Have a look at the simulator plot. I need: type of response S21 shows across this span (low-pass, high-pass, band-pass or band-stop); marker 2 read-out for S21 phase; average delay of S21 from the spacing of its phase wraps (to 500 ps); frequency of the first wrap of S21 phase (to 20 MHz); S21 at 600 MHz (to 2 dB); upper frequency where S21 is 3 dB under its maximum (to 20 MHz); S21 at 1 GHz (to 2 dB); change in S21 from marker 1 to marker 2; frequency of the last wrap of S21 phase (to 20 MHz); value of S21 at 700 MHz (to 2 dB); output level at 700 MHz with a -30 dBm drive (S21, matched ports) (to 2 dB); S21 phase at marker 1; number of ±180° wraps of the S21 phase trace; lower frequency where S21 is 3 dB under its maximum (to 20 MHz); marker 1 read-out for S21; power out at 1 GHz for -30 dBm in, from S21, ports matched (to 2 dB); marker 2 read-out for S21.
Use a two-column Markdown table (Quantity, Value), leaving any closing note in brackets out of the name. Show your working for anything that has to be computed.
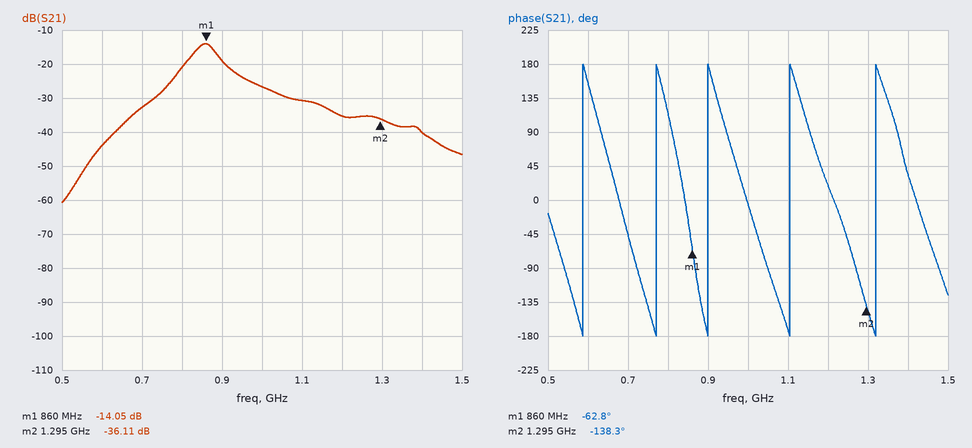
| Quantity | Value |
|---|---|
| type of response S21 shows across this span | band-pass |
| marker 2 read-out for S21 phase | -138.3° |
| average delay of S21 from the spacing of its phase wraps | 4 cycles / (1.32 GHz − 580 MHz) ≈ 5.41 ns, so 5.5 ns to the nearest 500 ps |
| frequency of the first wrap of S21 phase | 580 MHz |
| S21 at 600 MHz | -44 dB |
| upper frequency where S21 is 3 dB under its maximum | 880 MHz |
| S21 at 1 GHz | -26 dB |
| change in S21 from marker 1 to marker 2 | -36.11 − (-14.05) = -22.06 dB |
| frequency of the last wrap of S21 phase | 1.32 GHz |
| value of S21 at 700 MHz | -32 dB |
| output level at 700 MHz with a -30 dBm drive (S21, matched ports) | -30 dBm + (-32 dB) = -62 dBm |
| S21 phase at marker 1 | -62.8° |
| number of ±180° wraps of the S21 phase trace | 5 |
| lower frequency where S21 is 3 dB under its maximum | 820 MHz |
| marker 1 read-out for S21 | -14.05 dB |
| power out at 1 GHz for -30 dBm in, from S21, ports matched | -30 dBm + (-26 dB) = -56 dBm |
| marker 2 read-out for S21 | -36.11 dB |
